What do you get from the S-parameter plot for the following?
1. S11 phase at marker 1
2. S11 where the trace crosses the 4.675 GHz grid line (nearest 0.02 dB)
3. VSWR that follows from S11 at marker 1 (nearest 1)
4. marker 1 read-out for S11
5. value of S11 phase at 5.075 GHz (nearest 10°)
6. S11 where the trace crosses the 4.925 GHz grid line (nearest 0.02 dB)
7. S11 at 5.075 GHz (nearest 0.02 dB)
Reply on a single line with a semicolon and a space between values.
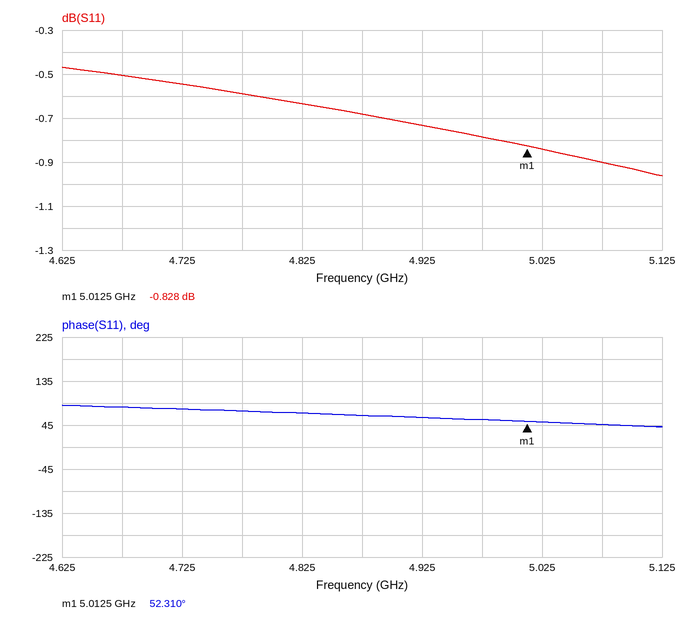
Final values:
52.310°; -0.50 dB; 21; -0.828 dB; 50°; -0.74 dB; -0.90 dB
